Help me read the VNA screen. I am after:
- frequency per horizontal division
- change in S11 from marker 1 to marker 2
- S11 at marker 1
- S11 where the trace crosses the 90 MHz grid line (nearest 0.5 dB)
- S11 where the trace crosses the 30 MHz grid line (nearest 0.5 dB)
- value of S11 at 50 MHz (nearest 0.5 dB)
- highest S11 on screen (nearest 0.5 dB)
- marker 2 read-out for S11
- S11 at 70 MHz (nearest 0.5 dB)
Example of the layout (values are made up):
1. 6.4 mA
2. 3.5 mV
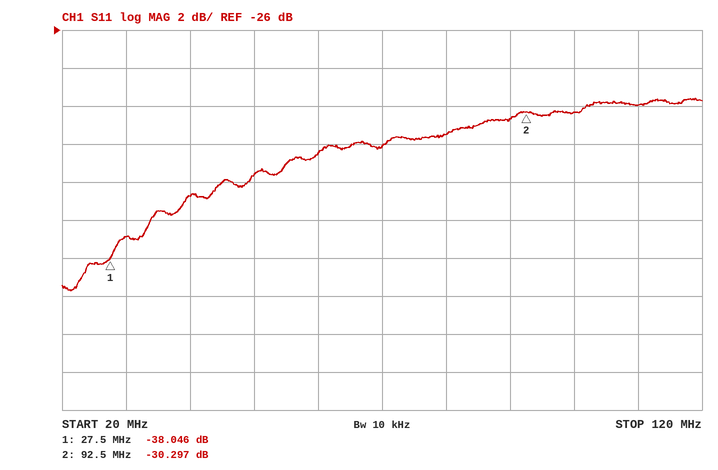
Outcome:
1. 10 MHz
2. 7.749 dB
3. -38.046 dB
4. -30.5 dB
5. -37.0 dB
6. -33.5 dB
7. -29.5 dB
8. -30.297 dB
9. -32.0 dB
